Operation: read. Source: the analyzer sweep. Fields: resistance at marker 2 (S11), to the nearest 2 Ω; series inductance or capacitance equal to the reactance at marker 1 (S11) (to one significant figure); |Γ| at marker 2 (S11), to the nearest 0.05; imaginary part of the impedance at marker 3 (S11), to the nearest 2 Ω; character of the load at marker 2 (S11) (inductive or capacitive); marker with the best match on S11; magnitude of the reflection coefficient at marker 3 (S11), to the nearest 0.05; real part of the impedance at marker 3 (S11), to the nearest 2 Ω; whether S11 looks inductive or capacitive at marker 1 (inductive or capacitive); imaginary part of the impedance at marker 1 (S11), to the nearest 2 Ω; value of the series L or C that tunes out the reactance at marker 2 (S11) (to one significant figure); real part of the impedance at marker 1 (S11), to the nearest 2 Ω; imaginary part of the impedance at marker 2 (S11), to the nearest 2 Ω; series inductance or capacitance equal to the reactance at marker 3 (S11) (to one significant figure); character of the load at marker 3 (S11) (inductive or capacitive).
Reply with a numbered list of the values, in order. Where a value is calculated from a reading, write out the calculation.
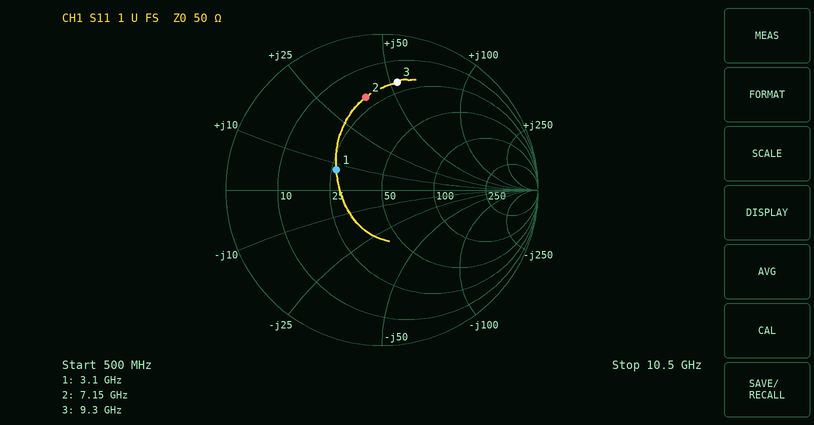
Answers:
1. 20 Ω
2. L = 8 Ω/(2π × 3.1 GHz) ≈ 411 pH, so 400 pH to one significant figure
3. 0.60
4. +54 Ω
5. inductive
6. marker 1
7. 0.70
8. 20 Ω
9. inductive
10. +8 Ω
11. C = 1/(2π × 7.15 GHz × 38 Ω) ≈ 586 fF, so 600 fF to one significant figure
12. 26 Ω
13. +38 Ω
14. L = 54 Ω/(2π × 9.3 GHz) ≈ 924 pH, so 900 pH to one significant figure
15. inductive
